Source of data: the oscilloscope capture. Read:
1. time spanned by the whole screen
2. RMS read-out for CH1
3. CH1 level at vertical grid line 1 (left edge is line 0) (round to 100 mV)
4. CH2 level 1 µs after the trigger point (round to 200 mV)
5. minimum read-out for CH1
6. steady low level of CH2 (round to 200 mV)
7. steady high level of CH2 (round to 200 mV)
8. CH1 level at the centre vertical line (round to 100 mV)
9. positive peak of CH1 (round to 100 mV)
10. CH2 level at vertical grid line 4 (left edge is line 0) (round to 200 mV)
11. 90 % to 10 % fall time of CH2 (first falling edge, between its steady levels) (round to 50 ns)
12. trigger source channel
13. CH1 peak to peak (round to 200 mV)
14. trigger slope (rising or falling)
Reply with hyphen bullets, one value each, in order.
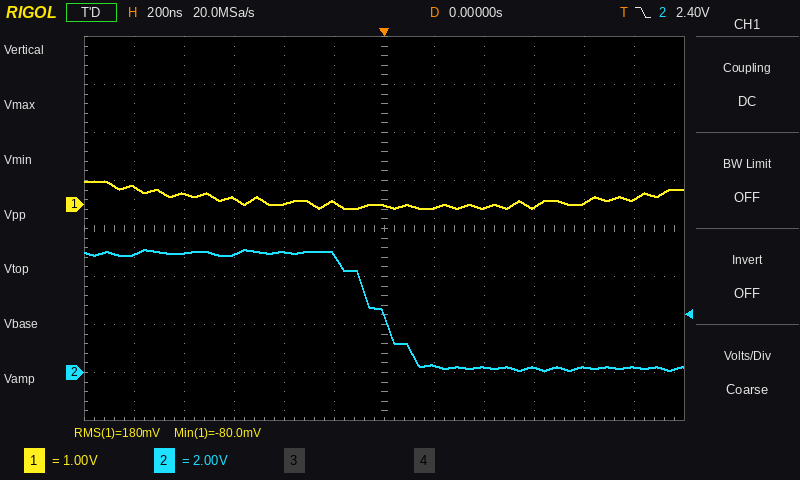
- 2.4 µs
- 180 mV
- 400 mV
- 200 mV
- -80.0 mV
- 200 mV
- 5.0 V
- 0.0 V
- 500 mV
- 5.0 V
- 300 ns
- CH2
- 600 mV
- falling
